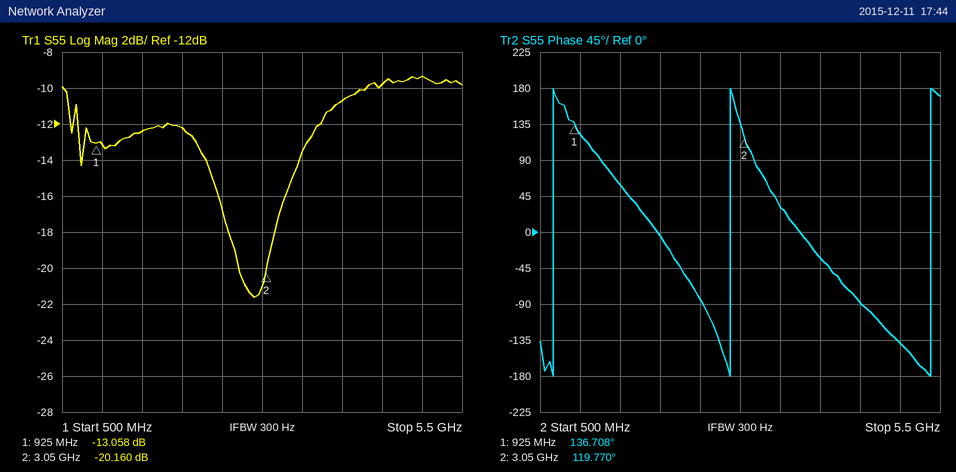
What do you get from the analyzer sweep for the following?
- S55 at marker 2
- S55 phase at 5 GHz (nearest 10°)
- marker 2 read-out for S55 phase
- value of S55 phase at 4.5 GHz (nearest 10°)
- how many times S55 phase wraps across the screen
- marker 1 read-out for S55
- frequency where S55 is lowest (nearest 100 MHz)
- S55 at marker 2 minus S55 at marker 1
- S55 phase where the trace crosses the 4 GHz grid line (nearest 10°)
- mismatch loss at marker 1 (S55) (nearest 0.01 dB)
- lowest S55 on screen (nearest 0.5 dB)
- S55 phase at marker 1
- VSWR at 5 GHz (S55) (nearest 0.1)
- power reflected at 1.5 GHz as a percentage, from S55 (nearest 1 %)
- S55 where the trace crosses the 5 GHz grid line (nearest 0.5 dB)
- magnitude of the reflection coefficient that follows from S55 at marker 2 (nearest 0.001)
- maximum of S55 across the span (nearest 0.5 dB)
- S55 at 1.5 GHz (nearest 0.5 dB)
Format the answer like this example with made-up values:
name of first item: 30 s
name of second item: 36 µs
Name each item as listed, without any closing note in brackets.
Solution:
S55 at marker 2: -20.160 dB
S55 phase at 5 GHz: -140°
marker 2 read-out for S55 phase: 119.770°
value of S55 phase at 4.5 GHz: -90°
how many times S55 phase wraps across the screen: 3
marker 1 read-out for S55: -13.058 dB
frequency where S55 is lowest: 2.9 GHz
S55 at marker 2 minus S55 at marker 1: -7.102 dB
S55 phase where the trace crosses the 4 GHz grid line: -30°
mismatch loss at marker 1 (S55): 0.22 dB
lowest S55 on screen: -21.5 dB
S55 phase at marker 1: 136.708°
VSWR at 5 GHz (S55): 2.0
power reflected at 1.5 GHz as a percentage, from S55: 6 %
S55 where the trace crosses the 5 GHz grid line: -9.5 dB
magnitude of the reflection coefficient that follows from S55 at marker 2: 0.098
maximum of S55 across the span: -9.5 dB
S55 at 1.5 GHz: -12.5 dB
